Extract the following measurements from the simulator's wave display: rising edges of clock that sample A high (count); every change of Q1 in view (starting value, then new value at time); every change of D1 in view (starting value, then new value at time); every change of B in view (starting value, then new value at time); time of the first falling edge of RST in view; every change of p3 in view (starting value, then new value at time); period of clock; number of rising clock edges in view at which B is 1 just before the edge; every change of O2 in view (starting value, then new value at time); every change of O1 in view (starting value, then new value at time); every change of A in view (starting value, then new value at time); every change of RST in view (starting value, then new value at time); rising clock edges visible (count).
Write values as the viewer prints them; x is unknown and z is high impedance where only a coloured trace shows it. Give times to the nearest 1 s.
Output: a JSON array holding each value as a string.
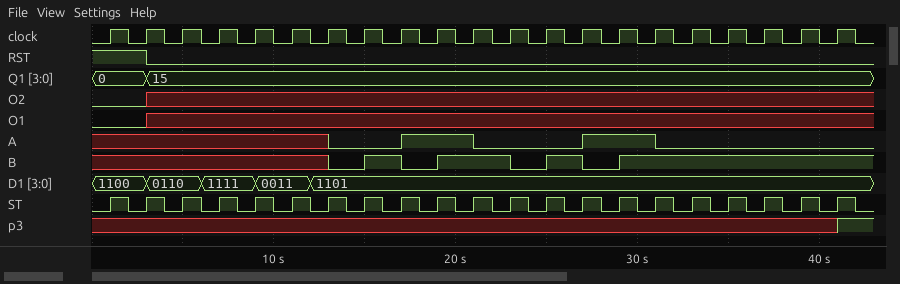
["4", "0, 15 at 3 s", "1100, 0110 at 3 s, 1111 at 6 s, 0011 at 9 s, 1101 at 12 s", "x, 0 at 13 s, 1 at 15 s, 0 at 17 s, 1 at 19 s, 0 at 23 s, 1 at 25 s, 0 at 27 s, 1 at 29 s", "3 s", "x, 1 at 41 s", "2 s", "10", "0, x at 3 s", "0, x at 3 s", "x, 0 at 13 s, 1 at 17 s, 0 at 21 s, 1 at 27 s, 0 at 31 s", "1, 0 at 3 s", "21"]
